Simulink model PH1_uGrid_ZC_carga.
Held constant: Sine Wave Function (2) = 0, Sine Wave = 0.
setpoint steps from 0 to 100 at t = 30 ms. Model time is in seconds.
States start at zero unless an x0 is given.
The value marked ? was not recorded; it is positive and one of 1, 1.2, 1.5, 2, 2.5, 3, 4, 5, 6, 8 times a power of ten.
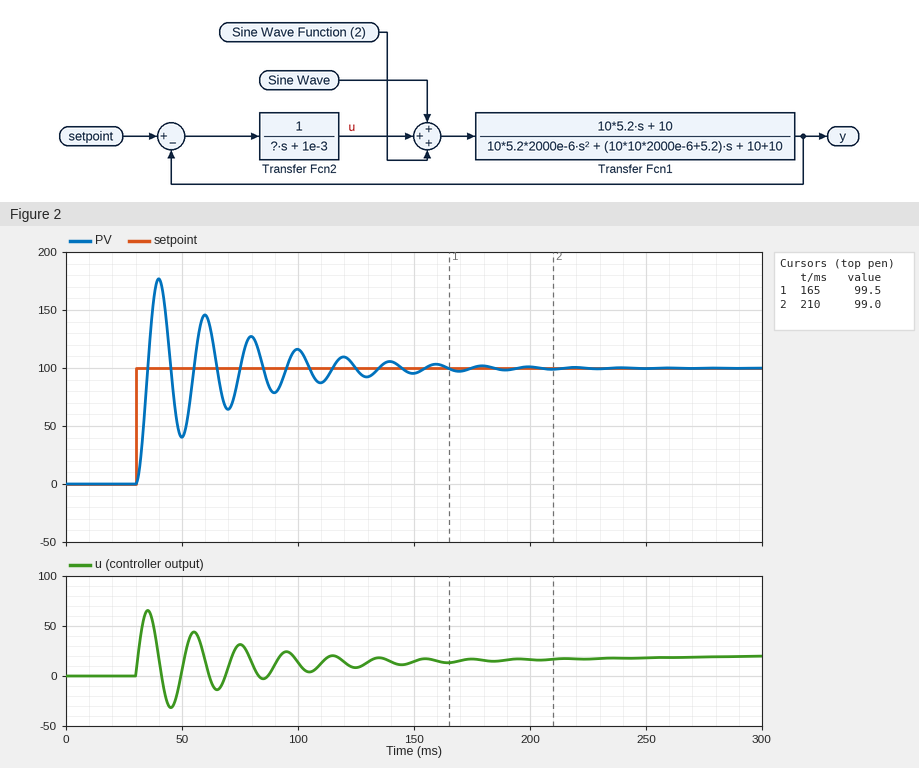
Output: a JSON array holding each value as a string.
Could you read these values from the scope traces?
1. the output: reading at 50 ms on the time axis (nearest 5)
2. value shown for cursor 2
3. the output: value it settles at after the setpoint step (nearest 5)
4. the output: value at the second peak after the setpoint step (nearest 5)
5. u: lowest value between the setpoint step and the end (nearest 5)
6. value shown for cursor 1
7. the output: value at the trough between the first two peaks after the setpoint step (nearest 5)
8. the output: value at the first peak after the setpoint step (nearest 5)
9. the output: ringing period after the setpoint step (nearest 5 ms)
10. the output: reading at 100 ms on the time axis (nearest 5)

["40", "99.0", "100", "145", "-30", "99.5", "40", "175", "20 ms", "115"]
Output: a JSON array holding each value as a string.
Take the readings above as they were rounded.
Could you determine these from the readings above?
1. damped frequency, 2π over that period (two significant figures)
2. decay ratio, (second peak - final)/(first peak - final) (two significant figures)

["0.31 rad/ms", "0.60"]
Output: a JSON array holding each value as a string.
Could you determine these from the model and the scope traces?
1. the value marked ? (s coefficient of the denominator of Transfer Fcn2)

["0.005"]
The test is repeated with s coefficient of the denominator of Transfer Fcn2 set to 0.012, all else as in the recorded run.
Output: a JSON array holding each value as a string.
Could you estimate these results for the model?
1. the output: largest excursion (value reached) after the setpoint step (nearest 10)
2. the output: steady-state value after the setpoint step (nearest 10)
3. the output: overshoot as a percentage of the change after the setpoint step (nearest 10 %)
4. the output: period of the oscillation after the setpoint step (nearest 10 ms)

["170", "100", "70 %", "30 ms"]
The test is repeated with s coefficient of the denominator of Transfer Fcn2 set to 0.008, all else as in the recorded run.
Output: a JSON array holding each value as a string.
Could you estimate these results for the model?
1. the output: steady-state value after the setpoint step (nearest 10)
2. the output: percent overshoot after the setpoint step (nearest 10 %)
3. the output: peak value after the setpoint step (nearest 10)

["100", "70 %", "170"]
